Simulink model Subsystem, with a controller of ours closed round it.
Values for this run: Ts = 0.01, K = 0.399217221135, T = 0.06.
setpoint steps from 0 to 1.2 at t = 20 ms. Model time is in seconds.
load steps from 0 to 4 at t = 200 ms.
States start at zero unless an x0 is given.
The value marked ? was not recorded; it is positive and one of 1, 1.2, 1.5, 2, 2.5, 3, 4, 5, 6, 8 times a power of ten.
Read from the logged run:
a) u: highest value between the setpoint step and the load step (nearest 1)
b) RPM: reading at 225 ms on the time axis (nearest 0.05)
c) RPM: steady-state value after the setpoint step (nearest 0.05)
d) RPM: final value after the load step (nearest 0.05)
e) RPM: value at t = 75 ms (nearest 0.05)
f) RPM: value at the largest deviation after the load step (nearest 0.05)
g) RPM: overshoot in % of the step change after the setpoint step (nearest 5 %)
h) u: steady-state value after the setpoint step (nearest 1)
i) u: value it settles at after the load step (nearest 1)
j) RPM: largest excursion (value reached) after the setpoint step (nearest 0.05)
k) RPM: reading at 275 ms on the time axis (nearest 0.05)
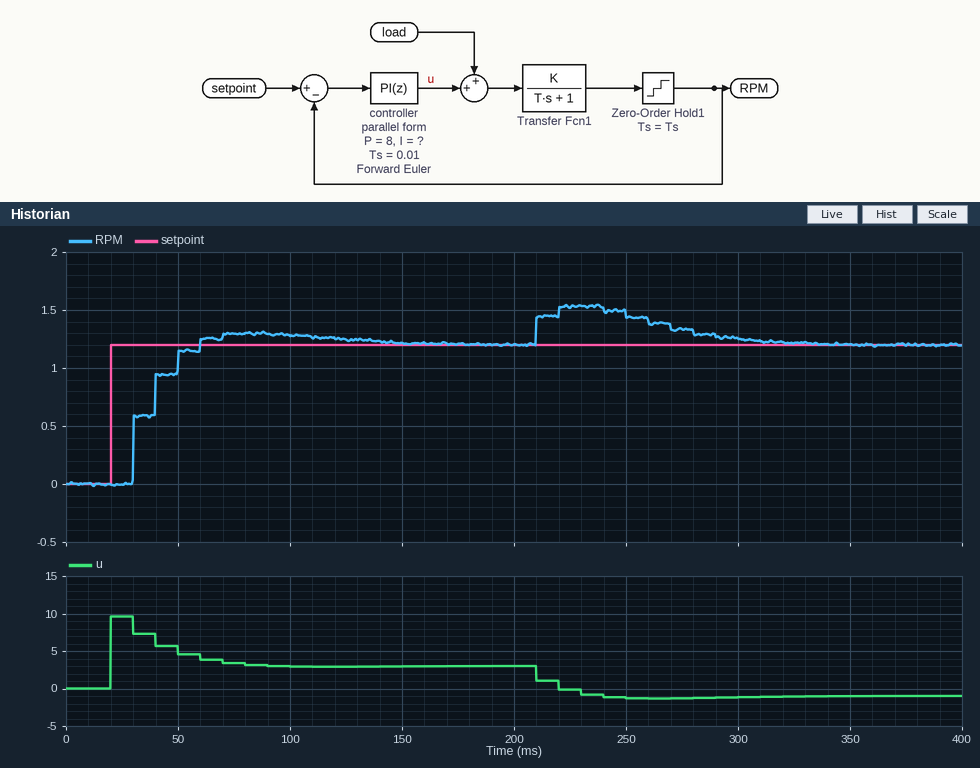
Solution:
10
1.55
1.20
1.20
1.30
1.55
10 %
3
-1
1.30
1.35
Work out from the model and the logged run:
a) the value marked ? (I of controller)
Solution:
200
